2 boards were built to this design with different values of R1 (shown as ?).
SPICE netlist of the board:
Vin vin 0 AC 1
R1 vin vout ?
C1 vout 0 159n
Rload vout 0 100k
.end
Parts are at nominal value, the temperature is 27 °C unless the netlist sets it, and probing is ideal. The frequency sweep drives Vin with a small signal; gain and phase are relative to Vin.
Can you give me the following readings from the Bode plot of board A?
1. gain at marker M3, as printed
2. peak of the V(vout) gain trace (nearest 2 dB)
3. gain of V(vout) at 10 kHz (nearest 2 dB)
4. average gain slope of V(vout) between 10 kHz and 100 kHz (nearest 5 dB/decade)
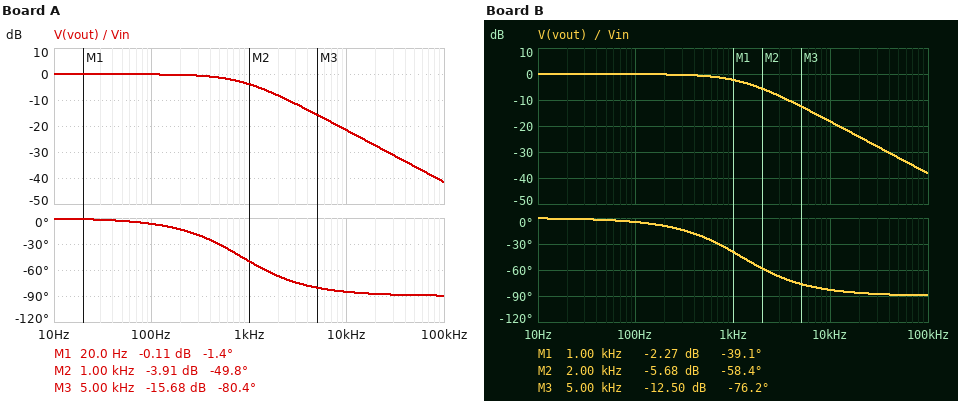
-15.68 dB
0 dB
-22 dB
-20 dB/decade
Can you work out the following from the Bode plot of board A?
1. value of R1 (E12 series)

1.2 kΩ
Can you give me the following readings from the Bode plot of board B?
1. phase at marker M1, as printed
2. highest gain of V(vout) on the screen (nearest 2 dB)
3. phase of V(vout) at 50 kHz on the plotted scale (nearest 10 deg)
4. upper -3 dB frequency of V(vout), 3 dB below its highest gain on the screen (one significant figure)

-39.1 deg
0 dB
-90 deg
1 kHz
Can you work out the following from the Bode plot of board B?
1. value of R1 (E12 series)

820 Ω
